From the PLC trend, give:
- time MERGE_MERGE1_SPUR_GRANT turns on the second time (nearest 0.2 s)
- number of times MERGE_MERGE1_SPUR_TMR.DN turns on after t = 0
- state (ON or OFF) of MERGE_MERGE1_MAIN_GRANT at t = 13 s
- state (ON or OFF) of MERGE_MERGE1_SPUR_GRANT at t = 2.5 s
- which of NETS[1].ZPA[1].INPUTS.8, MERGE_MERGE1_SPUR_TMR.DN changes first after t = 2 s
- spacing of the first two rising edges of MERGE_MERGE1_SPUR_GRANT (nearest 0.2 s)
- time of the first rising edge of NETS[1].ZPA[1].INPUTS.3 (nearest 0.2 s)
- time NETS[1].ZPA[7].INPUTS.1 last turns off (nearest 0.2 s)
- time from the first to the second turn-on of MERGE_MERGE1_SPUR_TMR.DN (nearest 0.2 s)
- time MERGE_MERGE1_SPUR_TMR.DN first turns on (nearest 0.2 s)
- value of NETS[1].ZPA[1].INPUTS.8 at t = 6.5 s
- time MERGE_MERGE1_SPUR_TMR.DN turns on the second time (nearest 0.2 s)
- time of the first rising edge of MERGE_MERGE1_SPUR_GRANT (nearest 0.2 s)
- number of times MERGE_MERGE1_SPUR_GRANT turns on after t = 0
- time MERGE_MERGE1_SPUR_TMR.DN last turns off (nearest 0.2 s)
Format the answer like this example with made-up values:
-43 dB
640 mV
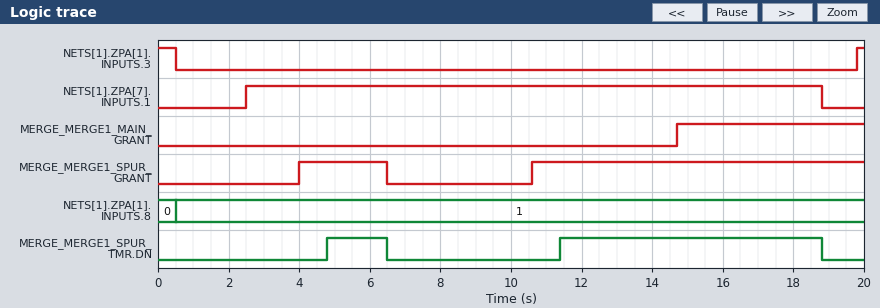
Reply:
10.6 s
2
OFF
OFF
MERGE_MERGE1_SPUR_TMR.DN
6.6 s
19.8 s
18.8 s
6.6 s
4.8 s
1
11.4 s
4.0 s
2
18.8 s
